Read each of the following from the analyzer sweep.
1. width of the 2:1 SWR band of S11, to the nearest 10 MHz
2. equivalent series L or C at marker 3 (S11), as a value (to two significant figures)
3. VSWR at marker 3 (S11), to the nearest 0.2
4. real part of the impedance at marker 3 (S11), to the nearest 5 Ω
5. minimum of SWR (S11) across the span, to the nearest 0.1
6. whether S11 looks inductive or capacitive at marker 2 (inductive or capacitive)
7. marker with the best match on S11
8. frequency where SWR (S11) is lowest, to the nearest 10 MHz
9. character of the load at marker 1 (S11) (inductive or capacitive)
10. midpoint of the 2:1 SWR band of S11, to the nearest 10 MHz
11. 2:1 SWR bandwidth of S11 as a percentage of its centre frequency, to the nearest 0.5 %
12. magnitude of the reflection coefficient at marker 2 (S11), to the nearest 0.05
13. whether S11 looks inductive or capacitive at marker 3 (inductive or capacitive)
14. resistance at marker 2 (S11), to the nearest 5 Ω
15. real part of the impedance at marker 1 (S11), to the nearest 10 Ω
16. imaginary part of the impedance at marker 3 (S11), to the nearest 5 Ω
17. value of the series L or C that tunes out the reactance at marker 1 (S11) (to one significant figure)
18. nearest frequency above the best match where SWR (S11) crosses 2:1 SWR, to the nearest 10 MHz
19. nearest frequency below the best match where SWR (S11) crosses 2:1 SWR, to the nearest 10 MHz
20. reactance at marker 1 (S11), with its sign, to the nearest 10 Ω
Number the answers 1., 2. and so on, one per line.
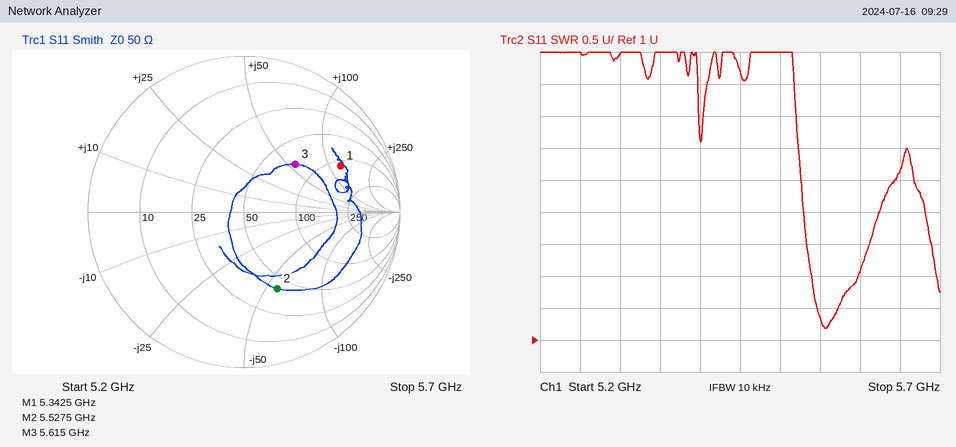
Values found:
1. 60 MHz
2. 1.6 nH
3. 2.6
4. 75 Ω
5. 1.2
6. capacitive
7. marker 3
8. 5.56 GHz
9. inductive
10. 5.57 GHz
11. 1.0 %
12. 0.55
13. inductive
14. 40 Ω
15. 110 Ω
16. +55 Ω
17. 200 fF
18. 5.60 GHz
19. 5.54 GHz
20. +130 Ω
